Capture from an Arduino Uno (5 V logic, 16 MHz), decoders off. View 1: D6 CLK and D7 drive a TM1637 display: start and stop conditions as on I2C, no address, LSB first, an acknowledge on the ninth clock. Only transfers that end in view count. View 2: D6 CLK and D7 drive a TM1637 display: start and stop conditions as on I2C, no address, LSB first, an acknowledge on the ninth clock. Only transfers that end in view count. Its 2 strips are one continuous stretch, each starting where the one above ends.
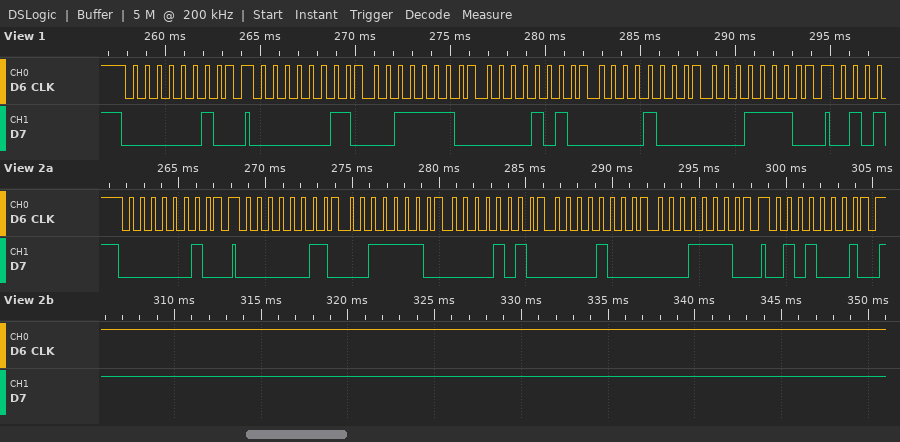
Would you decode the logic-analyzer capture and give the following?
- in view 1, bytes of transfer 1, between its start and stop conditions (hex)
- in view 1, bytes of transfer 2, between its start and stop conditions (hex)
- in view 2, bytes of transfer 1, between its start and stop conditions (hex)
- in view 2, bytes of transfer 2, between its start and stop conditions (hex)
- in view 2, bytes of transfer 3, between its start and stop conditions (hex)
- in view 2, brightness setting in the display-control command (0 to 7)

40
C0 7C 50 10 78
40
C0 7C 50 10 78
8A
2
